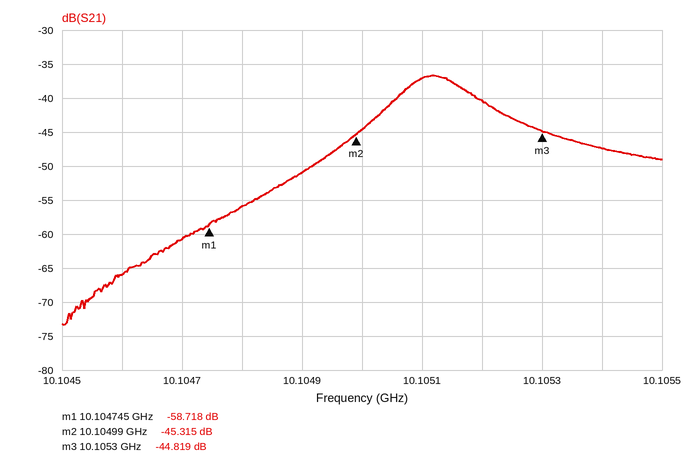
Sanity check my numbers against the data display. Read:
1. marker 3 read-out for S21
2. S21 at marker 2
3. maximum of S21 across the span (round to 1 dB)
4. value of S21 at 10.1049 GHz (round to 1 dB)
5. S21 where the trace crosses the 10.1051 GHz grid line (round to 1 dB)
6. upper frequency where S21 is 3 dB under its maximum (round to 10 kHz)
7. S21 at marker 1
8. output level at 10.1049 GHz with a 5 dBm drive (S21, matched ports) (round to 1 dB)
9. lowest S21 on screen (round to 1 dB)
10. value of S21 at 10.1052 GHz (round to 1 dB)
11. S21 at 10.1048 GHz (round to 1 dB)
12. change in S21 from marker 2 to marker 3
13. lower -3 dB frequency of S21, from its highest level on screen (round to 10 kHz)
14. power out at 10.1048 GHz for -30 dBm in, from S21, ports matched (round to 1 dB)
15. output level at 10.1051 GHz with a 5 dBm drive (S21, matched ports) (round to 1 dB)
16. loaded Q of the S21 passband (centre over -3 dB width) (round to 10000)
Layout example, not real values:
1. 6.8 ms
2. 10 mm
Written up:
1. -44.819 dB
2. -45.315 dB
3. -37 dB
4. -51 dB
5. -37 dB
6. 10.10519 GHz
7. -58.718 dB
8. -46 dBm
9. -73 dB
10. -40 dB
11. -56 dB
12. 0.496 dB
13. 10.10506 GHz
14. -86 dBm
15. -32 dBm
16. 80000
